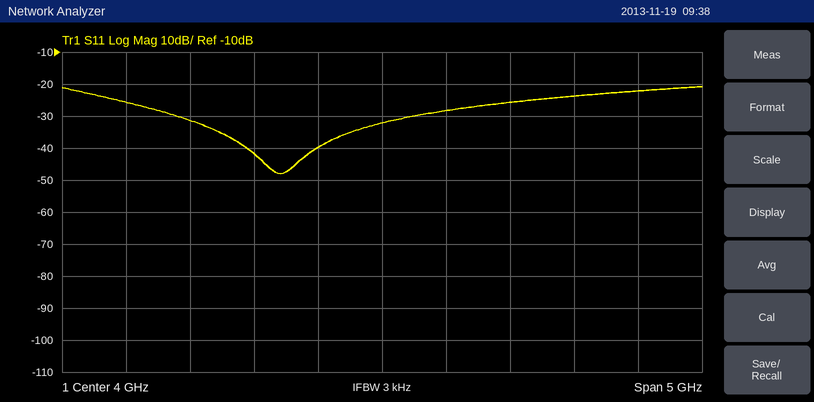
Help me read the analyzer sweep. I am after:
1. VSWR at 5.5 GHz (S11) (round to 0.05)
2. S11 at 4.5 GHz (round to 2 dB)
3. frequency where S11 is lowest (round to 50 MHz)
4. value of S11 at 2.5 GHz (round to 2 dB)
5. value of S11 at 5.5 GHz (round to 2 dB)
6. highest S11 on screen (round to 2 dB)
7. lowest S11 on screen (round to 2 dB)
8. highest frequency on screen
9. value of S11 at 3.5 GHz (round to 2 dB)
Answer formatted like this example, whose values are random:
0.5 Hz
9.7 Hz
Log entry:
1.15
-28 dB
3.20 GHz
-32 dB
-24 dB
-20 dB
-48 dB
6.5 GHz
-40 dB
